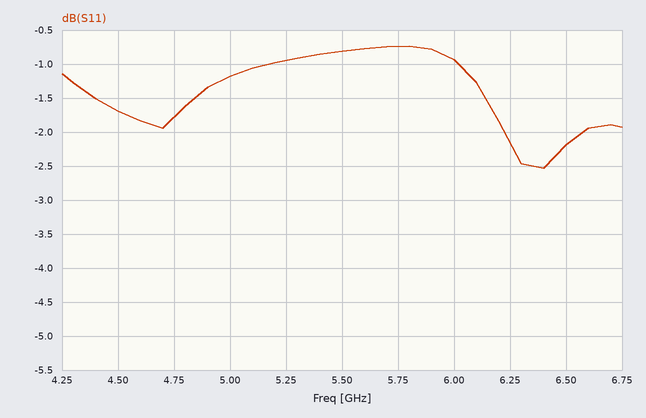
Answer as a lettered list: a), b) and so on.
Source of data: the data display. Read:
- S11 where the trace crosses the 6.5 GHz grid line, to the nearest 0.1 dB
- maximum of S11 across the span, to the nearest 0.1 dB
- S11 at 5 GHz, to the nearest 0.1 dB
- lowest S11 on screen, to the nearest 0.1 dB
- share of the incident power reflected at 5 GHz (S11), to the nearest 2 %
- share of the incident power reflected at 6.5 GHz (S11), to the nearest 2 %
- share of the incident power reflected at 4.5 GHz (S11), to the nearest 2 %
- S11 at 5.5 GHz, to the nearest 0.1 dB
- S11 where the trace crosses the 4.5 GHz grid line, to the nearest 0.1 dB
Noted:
a) -2.2 dB
b) -0.7 dB
c) -1.2 dB
d) -2.5 dB
e) 76 %
f) 60 %
g) 68 %
h) -0.8 dB
i) -1.7 dB
